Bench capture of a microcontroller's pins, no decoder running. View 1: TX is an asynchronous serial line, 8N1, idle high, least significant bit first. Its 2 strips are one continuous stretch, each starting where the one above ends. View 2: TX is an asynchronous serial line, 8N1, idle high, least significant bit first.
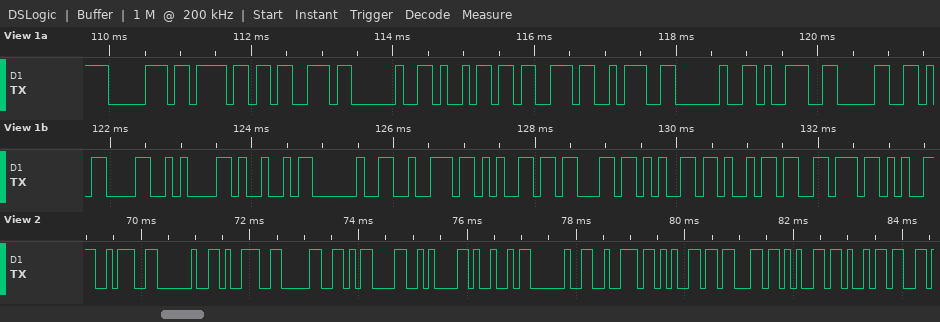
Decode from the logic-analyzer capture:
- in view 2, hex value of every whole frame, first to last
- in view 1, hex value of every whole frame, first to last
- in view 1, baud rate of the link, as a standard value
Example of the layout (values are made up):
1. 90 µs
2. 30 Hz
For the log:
1. 3A 20 39 30 0D 0A 49 20 72 65 63 65 69
2. 0x70 0x6F 0x73 0x20 0x69 0x73 0x3A 0x20 0x39 0x30 0x0D 0x0A 0x49 0x20 0x72 0x65 0x63 0x65 0x69 0x76
3. 9600 baud
